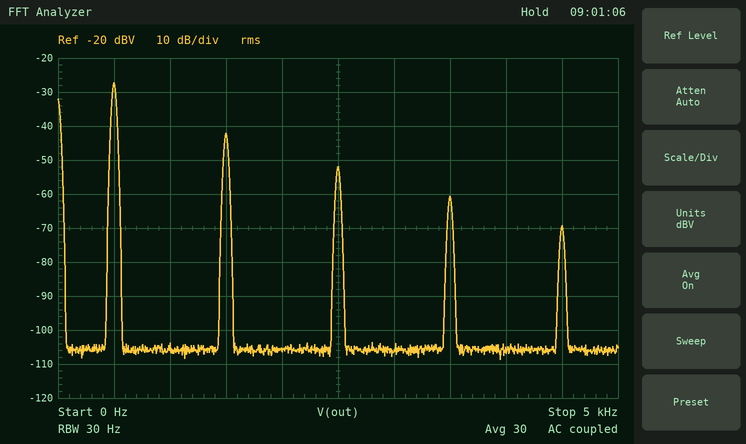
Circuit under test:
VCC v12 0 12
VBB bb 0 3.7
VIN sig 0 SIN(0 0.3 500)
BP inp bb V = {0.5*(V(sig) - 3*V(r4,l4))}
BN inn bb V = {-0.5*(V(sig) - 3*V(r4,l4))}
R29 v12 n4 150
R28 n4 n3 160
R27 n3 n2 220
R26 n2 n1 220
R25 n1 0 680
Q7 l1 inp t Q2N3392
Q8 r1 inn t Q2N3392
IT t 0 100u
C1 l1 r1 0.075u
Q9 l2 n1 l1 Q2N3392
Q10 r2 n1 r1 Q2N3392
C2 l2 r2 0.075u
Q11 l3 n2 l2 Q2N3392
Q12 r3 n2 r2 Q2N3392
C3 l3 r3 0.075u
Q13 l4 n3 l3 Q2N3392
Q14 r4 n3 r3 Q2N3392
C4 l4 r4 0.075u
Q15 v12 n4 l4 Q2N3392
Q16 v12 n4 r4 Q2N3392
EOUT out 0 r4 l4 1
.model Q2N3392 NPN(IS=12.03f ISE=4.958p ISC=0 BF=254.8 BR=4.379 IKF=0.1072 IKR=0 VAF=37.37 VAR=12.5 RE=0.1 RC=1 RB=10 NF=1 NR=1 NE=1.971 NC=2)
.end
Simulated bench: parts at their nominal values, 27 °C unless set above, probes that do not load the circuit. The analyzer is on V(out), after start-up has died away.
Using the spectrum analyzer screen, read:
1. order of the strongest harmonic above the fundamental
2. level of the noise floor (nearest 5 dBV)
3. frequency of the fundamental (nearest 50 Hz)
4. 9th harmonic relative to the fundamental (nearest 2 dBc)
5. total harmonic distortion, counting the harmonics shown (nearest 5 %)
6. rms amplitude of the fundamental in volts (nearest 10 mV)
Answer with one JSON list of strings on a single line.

["3", "-105 dBV", "500 Hz", "-42 dBc", "20 %", "40 mV"]
